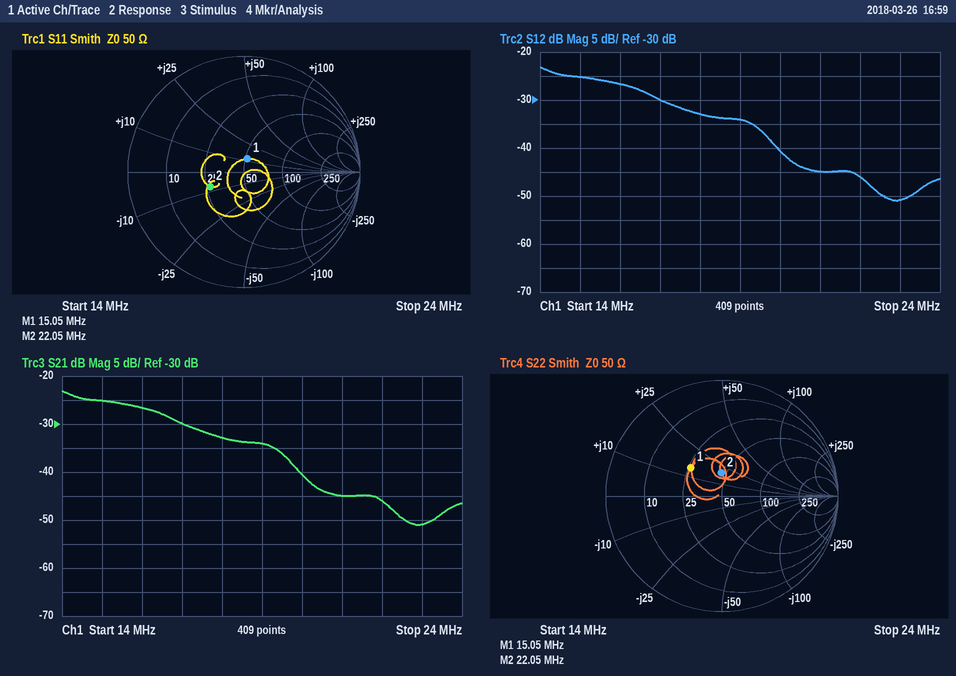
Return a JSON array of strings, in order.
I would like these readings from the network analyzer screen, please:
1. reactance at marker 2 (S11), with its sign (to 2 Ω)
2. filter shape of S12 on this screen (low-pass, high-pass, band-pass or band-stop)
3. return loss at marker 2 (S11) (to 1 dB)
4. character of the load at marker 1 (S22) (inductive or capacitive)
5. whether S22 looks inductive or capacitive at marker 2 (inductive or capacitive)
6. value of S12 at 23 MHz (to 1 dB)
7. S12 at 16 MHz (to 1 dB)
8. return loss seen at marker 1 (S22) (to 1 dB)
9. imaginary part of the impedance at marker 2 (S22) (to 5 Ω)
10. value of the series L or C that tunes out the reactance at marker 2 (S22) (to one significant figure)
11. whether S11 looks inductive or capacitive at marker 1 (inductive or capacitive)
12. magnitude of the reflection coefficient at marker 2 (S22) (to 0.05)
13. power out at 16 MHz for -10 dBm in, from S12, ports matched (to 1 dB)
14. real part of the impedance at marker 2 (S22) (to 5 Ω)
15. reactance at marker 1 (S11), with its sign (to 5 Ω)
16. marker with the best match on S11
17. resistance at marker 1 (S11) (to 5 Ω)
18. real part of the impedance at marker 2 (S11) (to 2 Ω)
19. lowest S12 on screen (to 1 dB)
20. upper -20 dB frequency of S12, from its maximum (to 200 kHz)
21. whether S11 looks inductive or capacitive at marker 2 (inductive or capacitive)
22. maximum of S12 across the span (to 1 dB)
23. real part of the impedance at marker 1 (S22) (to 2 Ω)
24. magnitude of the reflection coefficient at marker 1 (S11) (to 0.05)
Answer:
["-8 Ω", "low-pass", "10 dB", "inductive", "inductive", "-51 dB", "-27 dB", "9 dB", "+20 Ω", "400 pF", "inductive", "0.20", "-37 dBm", "45 Ω", "+10 Ω", "marker 1", "50 Ω", "26 Ω", "-51 dB", "20.4 MHz", "capacitive", "-23 dB", "26 Ω", "0.10"]
